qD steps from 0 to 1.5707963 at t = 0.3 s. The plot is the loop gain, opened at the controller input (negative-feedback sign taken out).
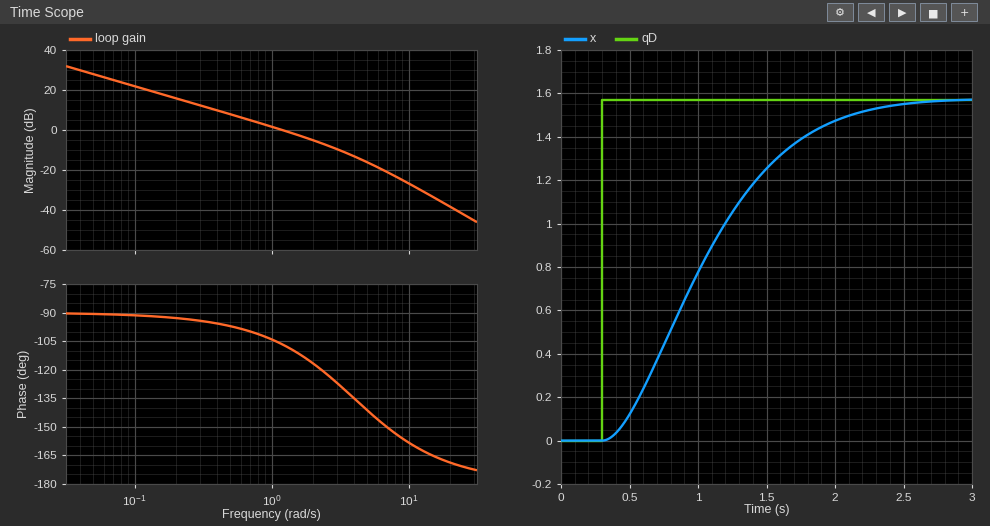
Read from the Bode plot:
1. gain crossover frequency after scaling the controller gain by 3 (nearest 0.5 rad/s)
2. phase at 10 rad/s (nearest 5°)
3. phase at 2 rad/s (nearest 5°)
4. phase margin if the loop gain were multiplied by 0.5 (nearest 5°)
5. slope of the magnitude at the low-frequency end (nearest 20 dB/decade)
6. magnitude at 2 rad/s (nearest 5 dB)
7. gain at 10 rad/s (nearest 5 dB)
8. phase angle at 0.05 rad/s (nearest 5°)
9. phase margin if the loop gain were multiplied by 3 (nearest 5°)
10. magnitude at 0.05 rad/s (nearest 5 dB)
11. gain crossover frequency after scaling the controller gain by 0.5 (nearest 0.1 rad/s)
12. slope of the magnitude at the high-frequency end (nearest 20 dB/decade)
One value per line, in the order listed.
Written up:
3.0 rad/s
-160°
-115°
80°
-20 dB/decade
-5 dB
-25 dB
-90°
55°
30 dB
0.6 rad/s
-40 dB/decade
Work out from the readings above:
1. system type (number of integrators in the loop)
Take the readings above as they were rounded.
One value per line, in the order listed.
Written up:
1
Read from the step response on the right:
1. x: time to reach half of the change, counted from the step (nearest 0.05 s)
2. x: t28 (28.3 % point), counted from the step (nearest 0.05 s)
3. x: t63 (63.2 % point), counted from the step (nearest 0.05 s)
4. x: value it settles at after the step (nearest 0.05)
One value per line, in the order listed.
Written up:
0.70 s
0.45 s
0.90 s
1.55
